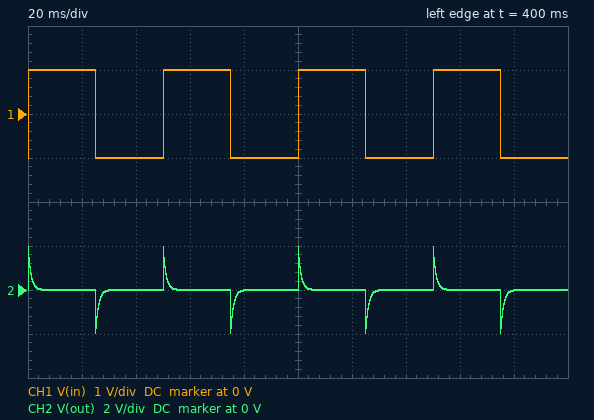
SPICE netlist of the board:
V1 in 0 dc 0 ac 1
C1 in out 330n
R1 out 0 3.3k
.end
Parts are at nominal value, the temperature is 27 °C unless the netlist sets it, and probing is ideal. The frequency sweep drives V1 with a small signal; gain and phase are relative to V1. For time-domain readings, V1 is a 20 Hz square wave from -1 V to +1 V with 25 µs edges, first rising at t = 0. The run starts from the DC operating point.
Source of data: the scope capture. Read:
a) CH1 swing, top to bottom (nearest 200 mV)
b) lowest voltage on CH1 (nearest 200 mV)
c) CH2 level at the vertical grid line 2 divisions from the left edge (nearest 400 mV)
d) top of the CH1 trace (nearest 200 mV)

2.0 V
-1.0 V
0 V
1.0 V
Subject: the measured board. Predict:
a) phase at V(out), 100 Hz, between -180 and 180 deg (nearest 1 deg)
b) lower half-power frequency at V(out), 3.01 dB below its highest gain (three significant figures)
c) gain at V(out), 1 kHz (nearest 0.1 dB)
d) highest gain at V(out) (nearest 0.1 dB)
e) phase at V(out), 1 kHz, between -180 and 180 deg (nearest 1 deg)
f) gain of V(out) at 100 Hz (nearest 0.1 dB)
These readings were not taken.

56 deg
146 Hz
-0.1 dB
0 dB
8 deg
-5.0 dB
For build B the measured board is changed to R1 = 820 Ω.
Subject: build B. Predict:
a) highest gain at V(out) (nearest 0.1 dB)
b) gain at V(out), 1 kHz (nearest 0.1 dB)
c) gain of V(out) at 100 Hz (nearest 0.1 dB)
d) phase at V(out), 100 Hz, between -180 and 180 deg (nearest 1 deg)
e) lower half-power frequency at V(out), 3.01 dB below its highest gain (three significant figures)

0 dB
-1.3 dB
-15.5 dB
80 deg
588 Hz
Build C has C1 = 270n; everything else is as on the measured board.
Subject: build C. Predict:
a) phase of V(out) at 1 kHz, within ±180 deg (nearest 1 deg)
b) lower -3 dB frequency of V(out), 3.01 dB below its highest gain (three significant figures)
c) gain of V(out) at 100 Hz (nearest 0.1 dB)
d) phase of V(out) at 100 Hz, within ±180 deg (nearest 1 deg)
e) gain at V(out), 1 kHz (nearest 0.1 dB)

10 deg
179 Hz
-6.2 dB
61 deg
-0.1 dB
